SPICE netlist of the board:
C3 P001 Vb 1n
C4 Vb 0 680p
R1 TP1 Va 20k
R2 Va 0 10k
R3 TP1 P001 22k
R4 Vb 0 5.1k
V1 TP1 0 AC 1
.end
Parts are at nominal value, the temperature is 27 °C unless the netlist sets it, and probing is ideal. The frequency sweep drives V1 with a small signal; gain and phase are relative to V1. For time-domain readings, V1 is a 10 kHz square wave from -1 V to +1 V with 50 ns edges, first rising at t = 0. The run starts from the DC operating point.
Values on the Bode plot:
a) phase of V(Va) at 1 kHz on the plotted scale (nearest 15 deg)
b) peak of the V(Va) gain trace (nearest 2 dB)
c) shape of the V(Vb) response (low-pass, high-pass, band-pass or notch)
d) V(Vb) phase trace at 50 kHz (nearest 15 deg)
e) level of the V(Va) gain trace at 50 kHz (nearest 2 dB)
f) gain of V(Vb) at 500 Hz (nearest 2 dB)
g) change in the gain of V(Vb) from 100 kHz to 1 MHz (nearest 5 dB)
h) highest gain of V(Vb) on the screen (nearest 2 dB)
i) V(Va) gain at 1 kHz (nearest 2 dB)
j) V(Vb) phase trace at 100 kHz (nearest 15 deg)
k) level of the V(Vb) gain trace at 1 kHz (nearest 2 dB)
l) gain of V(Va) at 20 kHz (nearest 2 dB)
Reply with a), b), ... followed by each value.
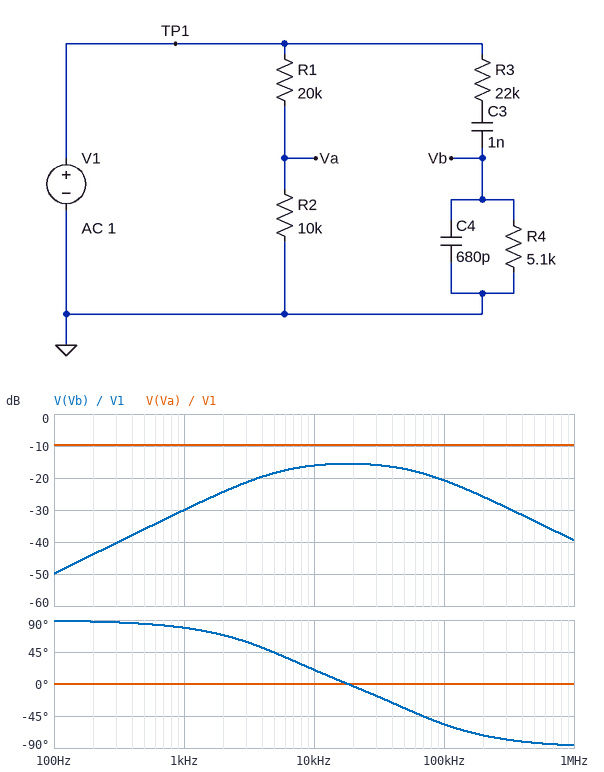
a) 0 deg
b) -10 dB
c) band-pass
d) -30 deg
e) -10 dB
f) -36 dB
g) -20 dB
h) -16 dB
i) -10 dB
j) -60 deg
k) -30 dB
l) -10 dB
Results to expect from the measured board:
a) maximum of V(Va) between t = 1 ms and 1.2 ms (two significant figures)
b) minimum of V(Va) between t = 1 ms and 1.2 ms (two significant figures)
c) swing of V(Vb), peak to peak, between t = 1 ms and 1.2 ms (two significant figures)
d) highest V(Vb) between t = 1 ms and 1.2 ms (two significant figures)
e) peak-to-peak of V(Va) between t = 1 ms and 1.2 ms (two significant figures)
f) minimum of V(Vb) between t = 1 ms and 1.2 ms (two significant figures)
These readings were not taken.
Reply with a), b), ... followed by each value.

a) 330 mV
b) -330 mV
c) 480 mV
d) 240 mV
e) 670 mV
f) -240 mV
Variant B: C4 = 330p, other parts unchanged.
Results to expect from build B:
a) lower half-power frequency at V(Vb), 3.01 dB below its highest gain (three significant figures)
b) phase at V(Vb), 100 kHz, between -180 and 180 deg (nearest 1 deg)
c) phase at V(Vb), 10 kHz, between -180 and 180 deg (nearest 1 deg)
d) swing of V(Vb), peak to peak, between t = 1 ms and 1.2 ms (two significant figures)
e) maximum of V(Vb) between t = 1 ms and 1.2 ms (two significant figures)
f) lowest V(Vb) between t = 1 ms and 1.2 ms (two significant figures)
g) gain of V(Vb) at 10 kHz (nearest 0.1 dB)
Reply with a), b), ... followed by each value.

a) 5.30 kHz
b) -37 deg
c) 25 deg
d) 540 mV
e) 270 mV
f) -270 mV
g) -15.9 dB
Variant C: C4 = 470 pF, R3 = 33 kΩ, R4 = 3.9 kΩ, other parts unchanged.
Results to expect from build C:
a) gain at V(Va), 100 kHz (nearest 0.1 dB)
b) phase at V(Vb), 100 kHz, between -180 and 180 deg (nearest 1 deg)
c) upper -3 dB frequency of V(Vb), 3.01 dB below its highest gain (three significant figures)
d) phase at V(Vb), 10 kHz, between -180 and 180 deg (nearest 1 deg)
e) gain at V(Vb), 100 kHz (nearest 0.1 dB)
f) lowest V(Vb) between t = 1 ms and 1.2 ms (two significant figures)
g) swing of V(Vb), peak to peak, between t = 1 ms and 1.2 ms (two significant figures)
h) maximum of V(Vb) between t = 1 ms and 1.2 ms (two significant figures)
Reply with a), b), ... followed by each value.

a) -9.5 dB
b) -43 deg
c) 106 kHz
d) 17 deg
e) -22.7 dB
f) -140 mV
g) 290 mV
h) 140 mV
